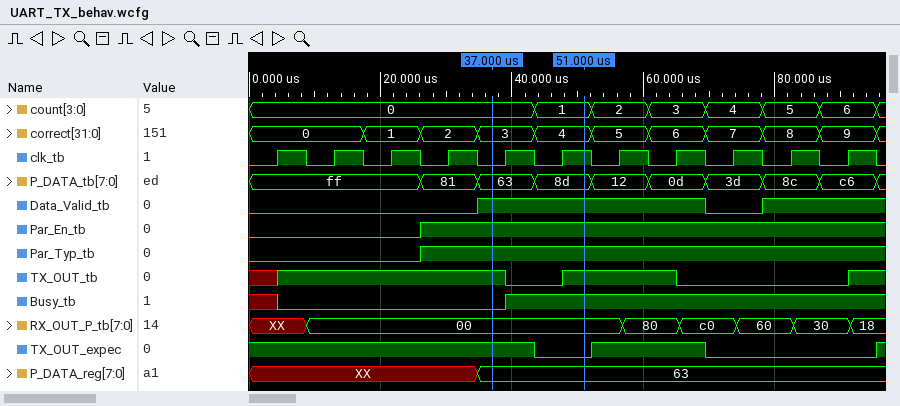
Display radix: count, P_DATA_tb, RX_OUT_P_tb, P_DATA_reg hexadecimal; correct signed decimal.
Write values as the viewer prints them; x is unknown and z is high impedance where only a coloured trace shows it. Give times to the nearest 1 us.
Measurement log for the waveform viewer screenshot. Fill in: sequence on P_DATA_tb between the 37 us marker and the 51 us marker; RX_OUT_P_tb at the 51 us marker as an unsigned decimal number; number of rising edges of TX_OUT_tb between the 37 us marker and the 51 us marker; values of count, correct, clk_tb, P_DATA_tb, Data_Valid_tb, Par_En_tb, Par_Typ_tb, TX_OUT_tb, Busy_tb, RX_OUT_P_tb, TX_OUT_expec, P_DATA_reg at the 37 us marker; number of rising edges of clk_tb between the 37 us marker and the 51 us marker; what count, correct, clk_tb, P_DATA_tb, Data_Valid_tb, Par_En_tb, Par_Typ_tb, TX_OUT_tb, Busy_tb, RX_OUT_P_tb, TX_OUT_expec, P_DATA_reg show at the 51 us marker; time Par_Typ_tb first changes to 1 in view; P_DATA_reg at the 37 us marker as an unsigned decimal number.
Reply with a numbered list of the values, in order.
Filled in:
1. 63, 8d
2. 0
3. 1
4. count=0, correct=3, clk_tb=0, P_DATA_tb=63, Data_Valid_tb=1, Par_En_tb=1, Par_Typ_tb=1, TX_OUT_tb=1, Busy_tb=0, RX_OUT_P_tb=00, TX_OUT_expec=1, P_DATA_reg=63
5. 2
6. count=1, correct=4, clk_tb=1, P_DATA_tb=8d, Data_Valid_tb=1, Par_En_tb=1, Par_Typ_tb=1, TX_OUT_tb=1, Busy_tb=1, RX_OUT_P_tb=00, TX_OUT_expec=0, P_DATA_reg=63
7. 26 us
8. 99
